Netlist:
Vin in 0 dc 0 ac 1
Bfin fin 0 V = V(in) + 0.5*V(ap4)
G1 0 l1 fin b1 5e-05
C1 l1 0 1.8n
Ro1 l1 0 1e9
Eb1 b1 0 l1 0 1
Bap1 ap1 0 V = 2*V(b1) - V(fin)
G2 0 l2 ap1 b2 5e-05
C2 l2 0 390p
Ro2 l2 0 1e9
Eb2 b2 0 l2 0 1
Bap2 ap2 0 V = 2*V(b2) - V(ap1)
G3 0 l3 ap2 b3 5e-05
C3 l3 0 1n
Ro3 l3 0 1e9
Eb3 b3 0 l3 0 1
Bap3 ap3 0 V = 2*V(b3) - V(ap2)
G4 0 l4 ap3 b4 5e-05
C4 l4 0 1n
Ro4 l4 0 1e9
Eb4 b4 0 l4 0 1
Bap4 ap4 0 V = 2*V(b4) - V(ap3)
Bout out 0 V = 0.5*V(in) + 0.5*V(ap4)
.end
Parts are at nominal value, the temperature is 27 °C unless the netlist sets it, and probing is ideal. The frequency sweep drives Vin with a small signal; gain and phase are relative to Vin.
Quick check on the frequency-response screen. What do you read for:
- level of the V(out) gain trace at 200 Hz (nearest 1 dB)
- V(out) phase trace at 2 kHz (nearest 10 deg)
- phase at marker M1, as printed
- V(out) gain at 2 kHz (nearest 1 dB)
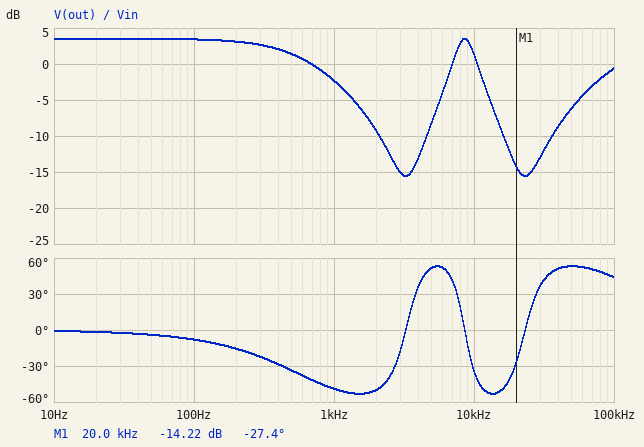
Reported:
3 dB
-50 deg
-27.4 deg
-9 dB
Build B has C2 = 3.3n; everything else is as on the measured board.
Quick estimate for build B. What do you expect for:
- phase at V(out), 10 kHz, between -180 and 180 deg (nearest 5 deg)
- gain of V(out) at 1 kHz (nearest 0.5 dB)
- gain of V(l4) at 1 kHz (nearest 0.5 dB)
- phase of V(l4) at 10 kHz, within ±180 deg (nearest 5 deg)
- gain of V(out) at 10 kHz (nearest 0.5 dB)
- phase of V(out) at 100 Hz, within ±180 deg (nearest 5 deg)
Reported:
-45 deg
-7.0 dB
-1.5 dB
-95 deg
-11.0 dB
-15 deg
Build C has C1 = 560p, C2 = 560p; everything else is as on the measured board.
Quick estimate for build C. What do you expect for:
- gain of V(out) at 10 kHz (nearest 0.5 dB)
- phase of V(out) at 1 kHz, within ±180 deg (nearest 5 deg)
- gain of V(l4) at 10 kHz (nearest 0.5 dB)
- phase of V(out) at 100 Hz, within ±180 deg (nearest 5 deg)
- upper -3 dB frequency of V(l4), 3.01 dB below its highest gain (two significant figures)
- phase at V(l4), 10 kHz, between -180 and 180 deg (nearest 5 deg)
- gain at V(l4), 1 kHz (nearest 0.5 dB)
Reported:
3.0 dB
-45 deg
1.5 dB
-5 deg
910 Hz
80 deg
2.5 dB
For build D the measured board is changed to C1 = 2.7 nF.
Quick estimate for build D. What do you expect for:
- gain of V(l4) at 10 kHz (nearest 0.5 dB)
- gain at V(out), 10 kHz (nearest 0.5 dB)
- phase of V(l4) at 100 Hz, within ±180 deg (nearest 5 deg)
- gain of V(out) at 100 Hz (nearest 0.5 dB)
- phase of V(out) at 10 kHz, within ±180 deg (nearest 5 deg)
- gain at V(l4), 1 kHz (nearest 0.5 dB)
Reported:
-1.5 dB
-0.5 dB
-15 deg
3.5 dB
-45 deg
0 dB
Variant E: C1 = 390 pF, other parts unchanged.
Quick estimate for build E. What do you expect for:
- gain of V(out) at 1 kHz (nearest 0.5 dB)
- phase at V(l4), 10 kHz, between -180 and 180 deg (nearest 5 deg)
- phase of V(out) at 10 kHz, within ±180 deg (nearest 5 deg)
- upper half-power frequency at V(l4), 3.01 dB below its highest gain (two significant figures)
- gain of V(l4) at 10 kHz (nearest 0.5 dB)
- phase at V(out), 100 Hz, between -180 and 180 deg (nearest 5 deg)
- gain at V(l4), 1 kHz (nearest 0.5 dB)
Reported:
0 dB
130 deg
45 deg
1.0 kHz
-2.0 dB
-5 deg
3.0 dB
